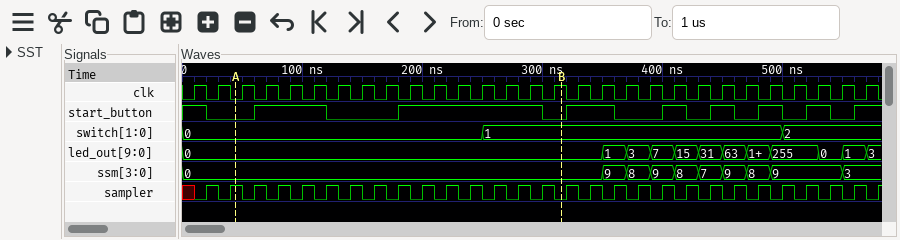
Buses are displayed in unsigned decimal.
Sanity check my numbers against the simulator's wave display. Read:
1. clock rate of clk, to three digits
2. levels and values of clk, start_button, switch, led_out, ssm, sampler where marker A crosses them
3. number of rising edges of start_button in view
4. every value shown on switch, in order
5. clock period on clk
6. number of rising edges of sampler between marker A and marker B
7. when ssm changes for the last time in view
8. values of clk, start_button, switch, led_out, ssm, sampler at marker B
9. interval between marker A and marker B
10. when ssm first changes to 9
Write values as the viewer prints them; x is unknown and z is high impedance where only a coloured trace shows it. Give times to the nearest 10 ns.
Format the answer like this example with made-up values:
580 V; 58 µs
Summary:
50.0 MHz; clk=0, start_button=0, switch=0, led_out=0, ssm=0, sampler=1; 8; 0, 1, 2; 20 ns; 13; 550 ns; clk=1, start_button=0, switch=1, led_out=0, ssm=0, sampler=0; 270 ns; 350 ns
